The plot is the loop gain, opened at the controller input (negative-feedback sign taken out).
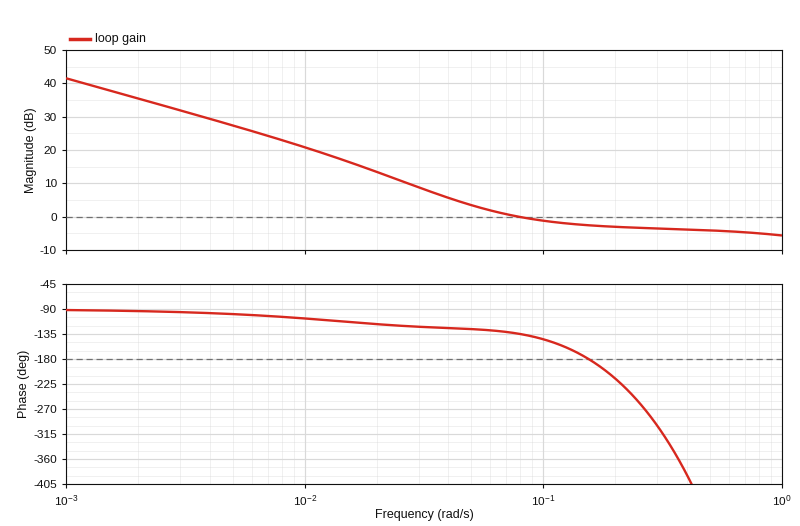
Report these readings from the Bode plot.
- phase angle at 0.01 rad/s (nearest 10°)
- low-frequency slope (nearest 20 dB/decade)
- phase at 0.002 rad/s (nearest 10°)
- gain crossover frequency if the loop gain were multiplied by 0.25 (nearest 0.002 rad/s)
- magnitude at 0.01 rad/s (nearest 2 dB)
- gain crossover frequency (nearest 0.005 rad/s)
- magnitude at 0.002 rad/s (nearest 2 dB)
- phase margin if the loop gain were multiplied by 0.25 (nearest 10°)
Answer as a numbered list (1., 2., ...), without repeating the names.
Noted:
1. -110°
2. -20 dB/decade
3. -90°
4. 0.022 rad/s
5. 20 dB
6. 0.080 rad/s
7. 36 dB
8. 60°
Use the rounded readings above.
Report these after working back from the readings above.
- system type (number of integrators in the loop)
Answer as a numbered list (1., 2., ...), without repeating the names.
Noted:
1. 1
